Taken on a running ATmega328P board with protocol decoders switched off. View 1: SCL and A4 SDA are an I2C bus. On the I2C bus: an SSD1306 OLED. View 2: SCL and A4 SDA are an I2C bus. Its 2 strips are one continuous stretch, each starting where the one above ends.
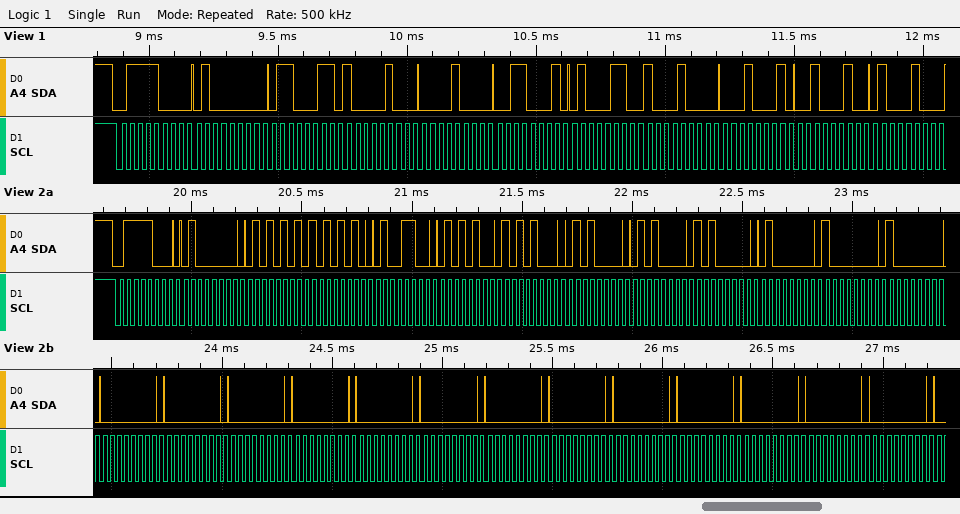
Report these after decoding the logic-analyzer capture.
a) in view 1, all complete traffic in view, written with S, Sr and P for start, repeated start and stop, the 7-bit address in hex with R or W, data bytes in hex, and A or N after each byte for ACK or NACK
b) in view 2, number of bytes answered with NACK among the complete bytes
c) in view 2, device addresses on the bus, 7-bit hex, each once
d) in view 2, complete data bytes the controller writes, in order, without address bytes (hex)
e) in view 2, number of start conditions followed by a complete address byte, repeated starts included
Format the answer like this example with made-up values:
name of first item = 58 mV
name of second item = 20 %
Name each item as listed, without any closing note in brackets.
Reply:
in view 1, all complete traffic in view, written with S, Sr and P for start, repeated start and stop, the 7-bit address in hex with R or W, data bytes in hex, and A or N after each byte for ACK or NACK = S 3CW A 40 A 63 A 84 A 08 A 31 A 46 A 88 A 11 A 22 A 44 A
in view 2, number of bytes answered with NACK among the complete bytes = 0
in view 2, device addresses on the bus, 7-bit hex, each once = 0x3C
in view 2, complete data bytes the controller writes, in order, without address bytes = 40 55 AA 4C 54 A8 50 50 A0 40 80 80 00 00 00 00 00 00 00 00 00 00 00 00 00
in view 2, number of start conditions followed by a complete address byte, repeated starts included = 1
